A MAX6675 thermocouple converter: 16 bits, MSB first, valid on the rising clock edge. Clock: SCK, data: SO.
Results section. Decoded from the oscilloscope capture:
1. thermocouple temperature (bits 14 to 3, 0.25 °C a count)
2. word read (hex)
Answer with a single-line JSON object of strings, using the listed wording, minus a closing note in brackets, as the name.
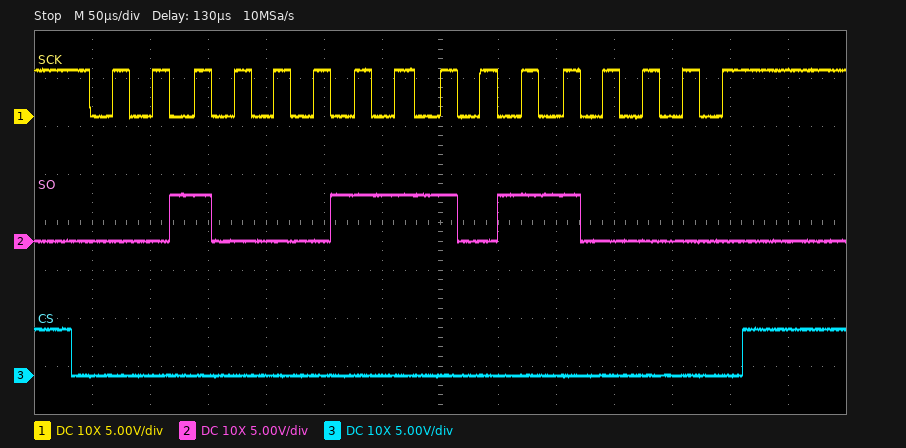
{"thermocouple temperature": "285.50 °C", "word read": "0x23B0"}
